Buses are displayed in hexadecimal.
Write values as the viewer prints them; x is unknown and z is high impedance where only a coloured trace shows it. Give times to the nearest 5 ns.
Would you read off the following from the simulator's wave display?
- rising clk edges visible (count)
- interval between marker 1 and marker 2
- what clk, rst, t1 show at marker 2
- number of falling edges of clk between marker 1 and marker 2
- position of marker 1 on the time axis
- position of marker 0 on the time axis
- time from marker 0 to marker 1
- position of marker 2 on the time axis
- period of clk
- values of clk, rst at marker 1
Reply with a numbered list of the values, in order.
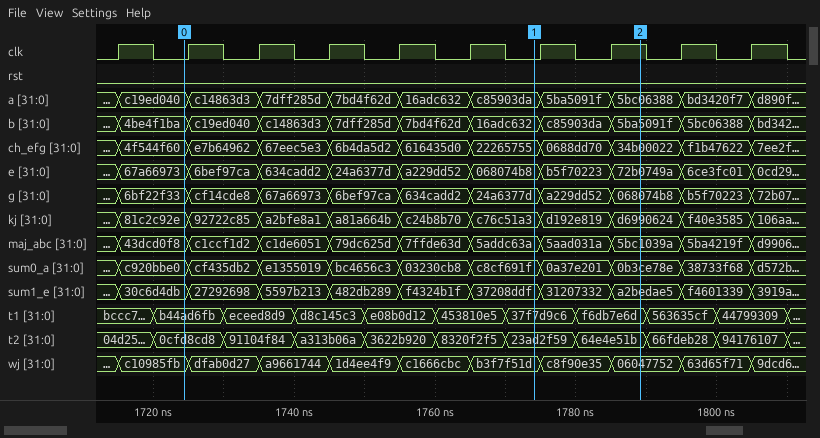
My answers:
1. 10
2. 15 ns
3. clk=1, rst=0, t1=f6db7e6d
4. 1
5. 1775 ns
6. 1725 ns
7. 50 ns
8. 1790 ns
9. 10 ns
10. clk=0, rst=0
